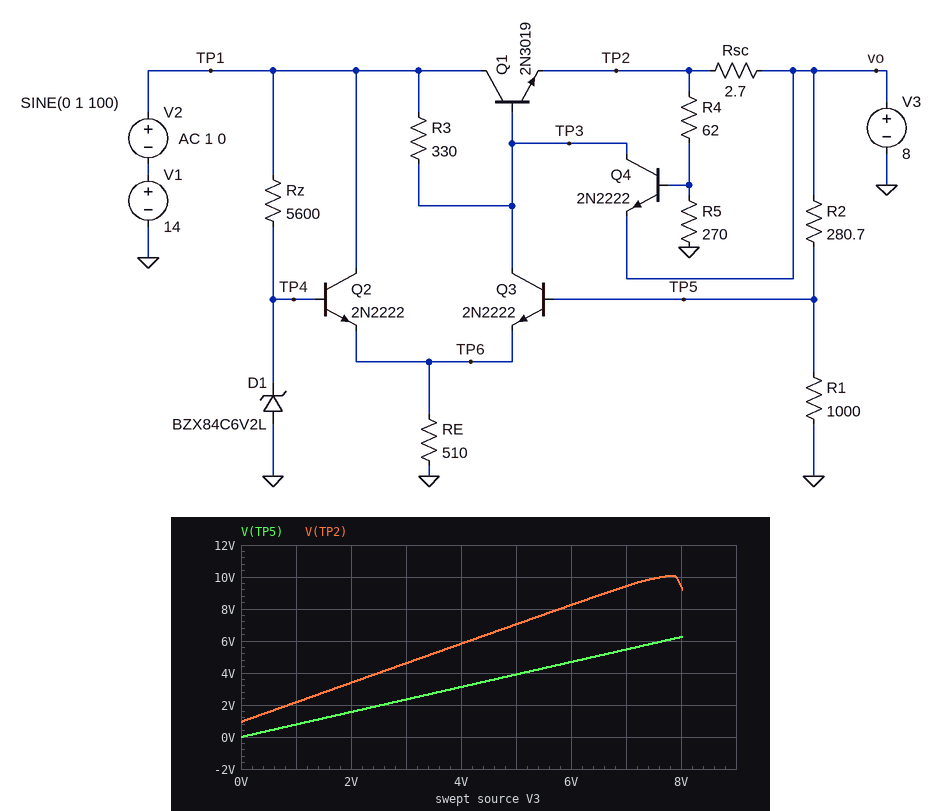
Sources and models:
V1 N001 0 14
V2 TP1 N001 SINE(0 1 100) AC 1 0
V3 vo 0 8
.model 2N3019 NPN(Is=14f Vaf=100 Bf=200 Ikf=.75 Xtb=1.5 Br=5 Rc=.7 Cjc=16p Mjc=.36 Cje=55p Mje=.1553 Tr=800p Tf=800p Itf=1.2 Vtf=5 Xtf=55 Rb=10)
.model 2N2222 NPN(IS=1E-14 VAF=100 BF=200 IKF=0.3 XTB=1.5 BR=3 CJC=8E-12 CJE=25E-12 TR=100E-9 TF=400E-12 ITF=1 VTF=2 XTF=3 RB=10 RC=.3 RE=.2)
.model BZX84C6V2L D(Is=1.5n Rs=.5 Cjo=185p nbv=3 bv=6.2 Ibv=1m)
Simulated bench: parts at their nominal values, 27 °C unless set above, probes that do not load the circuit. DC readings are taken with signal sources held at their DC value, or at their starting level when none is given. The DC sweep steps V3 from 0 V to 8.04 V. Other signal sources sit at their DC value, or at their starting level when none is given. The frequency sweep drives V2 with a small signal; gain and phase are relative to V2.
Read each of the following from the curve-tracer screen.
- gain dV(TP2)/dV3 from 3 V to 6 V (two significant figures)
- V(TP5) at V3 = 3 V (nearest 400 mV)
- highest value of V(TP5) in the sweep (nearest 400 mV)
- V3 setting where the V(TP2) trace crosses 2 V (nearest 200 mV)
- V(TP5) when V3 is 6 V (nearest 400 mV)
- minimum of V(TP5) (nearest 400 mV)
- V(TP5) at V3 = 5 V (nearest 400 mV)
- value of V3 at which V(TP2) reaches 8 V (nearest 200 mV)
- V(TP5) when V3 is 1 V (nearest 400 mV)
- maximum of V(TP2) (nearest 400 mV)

1.2 V/V
2.4 V
6.4 V
800 mV
4.8 V
0 V
4.0 V
5.8 V
800 mV
10.0 V
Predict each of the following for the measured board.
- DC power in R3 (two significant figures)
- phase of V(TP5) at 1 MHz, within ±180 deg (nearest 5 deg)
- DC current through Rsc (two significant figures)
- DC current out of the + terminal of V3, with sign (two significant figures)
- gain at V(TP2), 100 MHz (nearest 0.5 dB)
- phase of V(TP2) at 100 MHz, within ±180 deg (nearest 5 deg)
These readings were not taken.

42 mW
45 deg
530 mA
-520 mA
-21.5 dB
5 deg
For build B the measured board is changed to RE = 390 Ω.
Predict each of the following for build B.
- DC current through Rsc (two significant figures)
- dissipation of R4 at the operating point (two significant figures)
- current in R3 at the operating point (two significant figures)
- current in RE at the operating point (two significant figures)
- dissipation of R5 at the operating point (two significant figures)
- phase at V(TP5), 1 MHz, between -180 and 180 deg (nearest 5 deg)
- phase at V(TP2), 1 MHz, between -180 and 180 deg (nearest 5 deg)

440 mA
47 mW
12 mA
14 mA
210 mW
40 deg
-50 deg
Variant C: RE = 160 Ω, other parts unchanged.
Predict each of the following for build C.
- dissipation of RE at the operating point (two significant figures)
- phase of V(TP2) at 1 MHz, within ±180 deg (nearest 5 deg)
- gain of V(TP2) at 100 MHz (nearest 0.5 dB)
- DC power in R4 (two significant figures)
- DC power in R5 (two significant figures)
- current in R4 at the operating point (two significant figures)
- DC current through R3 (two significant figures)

190 mW
60 deg
-39.0 dB
35 mW
150 mW
24 mA
18 mA
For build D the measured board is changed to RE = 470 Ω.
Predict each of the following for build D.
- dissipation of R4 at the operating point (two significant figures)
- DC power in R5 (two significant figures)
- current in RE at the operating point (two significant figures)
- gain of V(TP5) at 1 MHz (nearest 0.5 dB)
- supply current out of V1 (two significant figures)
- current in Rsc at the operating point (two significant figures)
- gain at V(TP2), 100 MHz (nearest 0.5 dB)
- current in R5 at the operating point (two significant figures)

49 mW
210 mW
12 mA
-53.5 dB
540 mA
500 mA
-22.0 dB
28 mA
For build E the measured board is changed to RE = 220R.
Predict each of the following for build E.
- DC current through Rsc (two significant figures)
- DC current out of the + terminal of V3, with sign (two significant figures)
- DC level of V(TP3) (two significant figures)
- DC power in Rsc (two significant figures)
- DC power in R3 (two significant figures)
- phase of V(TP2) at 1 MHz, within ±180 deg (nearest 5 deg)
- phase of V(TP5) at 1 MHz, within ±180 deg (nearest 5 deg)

130 mA
-120 mA
9.1 V
46 mW
72 mW
-45 deg
35 deg
